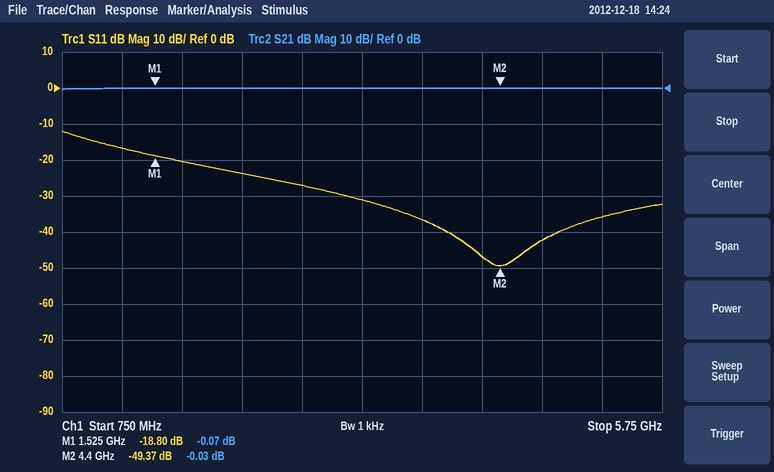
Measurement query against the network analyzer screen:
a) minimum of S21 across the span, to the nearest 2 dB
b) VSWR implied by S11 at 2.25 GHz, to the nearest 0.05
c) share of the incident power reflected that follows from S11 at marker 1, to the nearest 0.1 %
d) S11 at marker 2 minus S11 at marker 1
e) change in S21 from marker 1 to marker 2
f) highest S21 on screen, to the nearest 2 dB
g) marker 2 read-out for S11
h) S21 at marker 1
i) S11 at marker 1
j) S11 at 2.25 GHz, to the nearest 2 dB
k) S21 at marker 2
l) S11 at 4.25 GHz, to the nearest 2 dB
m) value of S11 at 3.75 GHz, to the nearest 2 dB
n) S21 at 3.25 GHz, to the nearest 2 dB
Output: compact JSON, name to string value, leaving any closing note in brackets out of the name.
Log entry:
{"minimum of S21 across the span, to the nearest 2 dB": "0 dB", "VSWR implied by S11 at 2.25 GHz, to the nearest 0.05": "1.15", "share of the incident power reflected that follows from S11 at marker 1, to the nearest 0.1 %": "1.3 %", "S11 at marker 2 minus S11 at marker 1": "-30.57 dB", "change in S21 from marker 1 to marker 2": "0.04 dB", "highest S21 on screen, to the nearest 2 dB": "0 dB", "marker 2 read-out for S11": "-49.37 dB", "S21 at marker 1": "-0.07 dB", "S11 at marker 1": "-18.80 dB", "S11 at 2.25 GHz, to the nearest 2 dB": "-24 dB", "S21 at marker 2": "-0.03 dB", "S11 at 4.25 GHz, to the nearest 2 dB": "-46 dB", "value of S11 at 3.75 GHz, to the nearest 2 dB": "-36 dB", "S21 at 3.25 GHz, to the nearest 2 dB": "0 dB"}
